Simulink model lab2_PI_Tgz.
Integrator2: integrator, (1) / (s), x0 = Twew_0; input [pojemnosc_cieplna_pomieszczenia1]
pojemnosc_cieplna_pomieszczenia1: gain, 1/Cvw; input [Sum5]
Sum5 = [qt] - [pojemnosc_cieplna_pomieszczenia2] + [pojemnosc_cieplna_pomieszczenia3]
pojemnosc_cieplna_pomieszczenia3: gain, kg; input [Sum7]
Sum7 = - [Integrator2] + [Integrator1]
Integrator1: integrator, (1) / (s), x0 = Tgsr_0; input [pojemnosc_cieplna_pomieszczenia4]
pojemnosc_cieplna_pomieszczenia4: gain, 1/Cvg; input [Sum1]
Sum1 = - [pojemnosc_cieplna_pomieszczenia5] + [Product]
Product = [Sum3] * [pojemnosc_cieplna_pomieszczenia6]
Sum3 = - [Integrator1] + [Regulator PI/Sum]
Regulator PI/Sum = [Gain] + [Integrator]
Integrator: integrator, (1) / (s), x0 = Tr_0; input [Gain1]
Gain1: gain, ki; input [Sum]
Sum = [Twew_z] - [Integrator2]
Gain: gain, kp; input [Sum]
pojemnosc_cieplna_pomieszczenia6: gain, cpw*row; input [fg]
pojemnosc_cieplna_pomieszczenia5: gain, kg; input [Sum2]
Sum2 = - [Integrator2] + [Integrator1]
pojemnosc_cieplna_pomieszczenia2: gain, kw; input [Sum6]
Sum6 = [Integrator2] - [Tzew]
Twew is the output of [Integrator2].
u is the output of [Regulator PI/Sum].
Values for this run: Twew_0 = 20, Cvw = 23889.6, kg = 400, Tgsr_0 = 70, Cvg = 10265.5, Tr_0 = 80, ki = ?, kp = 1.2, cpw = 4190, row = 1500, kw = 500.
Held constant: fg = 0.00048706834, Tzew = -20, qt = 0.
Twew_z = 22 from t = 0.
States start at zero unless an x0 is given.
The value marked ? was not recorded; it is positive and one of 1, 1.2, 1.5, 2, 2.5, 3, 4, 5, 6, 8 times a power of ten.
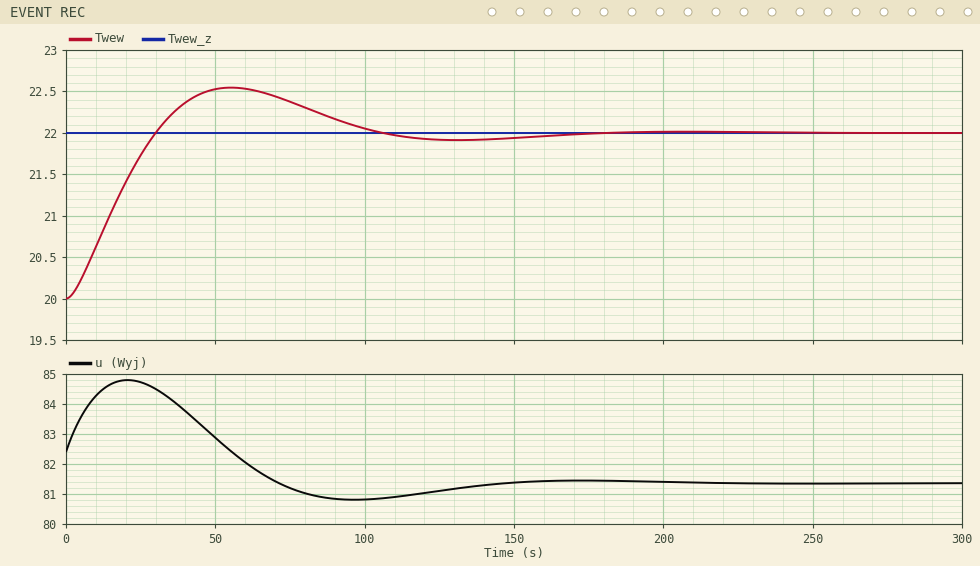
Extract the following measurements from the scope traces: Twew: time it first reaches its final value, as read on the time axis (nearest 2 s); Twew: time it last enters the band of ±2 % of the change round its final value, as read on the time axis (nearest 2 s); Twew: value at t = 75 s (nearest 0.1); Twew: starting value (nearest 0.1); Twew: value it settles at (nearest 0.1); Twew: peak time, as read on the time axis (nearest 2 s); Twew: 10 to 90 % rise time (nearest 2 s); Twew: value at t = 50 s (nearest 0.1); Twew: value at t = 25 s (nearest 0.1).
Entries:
30 s
160 s
22.4
20.0
22.0
56 s
22 s
22.5
21.7
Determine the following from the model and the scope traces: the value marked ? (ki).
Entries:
0.15
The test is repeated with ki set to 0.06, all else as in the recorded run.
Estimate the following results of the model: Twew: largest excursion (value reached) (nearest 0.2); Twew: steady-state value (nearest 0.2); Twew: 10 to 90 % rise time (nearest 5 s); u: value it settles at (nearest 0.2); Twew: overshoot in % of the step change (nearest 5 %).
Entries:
22.2
22.0
35 s
81.4
10 %
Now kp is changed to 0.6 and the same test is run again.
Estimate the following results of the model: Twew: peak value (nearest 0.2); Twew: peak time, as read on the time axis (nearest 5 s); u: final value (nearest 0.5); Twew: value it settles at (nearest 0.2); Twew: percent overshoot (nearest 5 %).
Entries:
22.6
60 s
81.5
22.0
35 %
